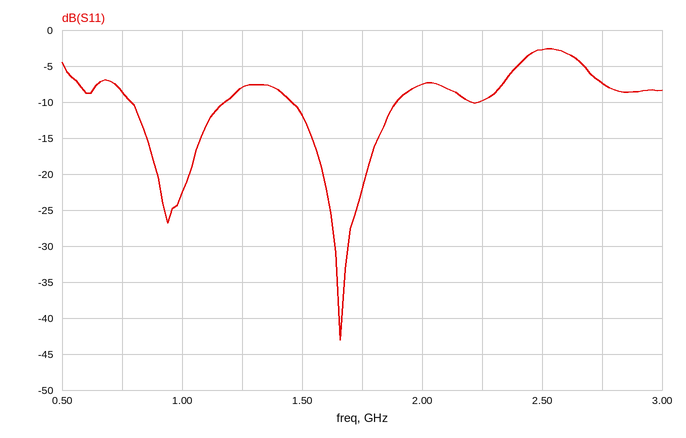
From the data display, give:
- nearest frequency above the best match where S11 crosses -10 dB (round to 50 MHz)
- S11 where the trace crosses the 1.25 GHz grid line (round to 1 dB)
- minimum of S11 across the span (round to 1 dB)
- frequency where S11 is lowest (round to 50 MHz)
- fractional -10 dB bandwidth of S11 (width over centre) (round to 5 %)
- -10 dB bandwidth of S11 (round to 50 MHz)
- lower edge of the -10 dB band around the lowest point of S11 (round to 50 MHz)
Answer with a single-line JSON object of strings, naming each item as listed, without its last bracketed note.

{"nearest frequency above the best match where S11 crosses -10 dB": "1.90 GHz", "S11 where the trace crosses the 1.25 GHz grid line": "-8 dB", "minimum of S11 across the span": "-43 dB", "frequency where S11 is lowest": "1.65 GHz", "fractional -10 dB bandwidth of S11 (width over centre)": "25 %", "-10 dB bandwidth of S11": "450 MHz", "lower edge of the -10 dB band around the lowest point of S11": "1.45 GHz"}
